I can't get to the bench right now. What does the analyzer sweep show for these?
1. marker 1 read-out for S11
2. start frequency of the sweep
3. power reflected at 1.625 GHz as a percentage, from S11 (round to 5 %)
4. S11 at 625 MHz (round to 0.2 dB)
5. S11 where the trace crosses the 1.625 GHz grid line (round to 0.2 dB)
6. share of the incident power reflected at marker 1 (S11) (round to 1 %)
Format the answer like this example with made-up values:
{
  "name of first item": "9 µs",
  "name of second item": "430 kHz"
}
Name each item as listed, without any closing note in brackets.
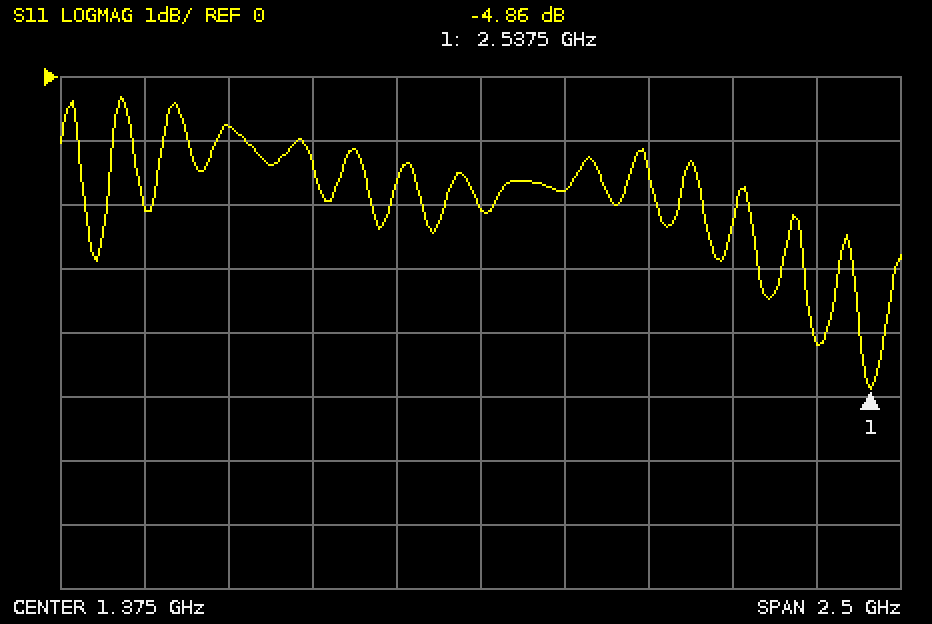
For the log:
{
  "marker 1 read-out for S11": "-4.86 dB",
  "start frequency of the sweep": "125 MHz",
  "power reflected at 1.625 GHz as a percentage, from S11": "65 %",
  "S11 at 625 MHz": "-0.8 dB",
  "S11 where the trace crosses the 1.625 GHz grid line": "-1.8 dB",
  "share of the incident power reflected at marker 1 (S11)": "33 %"
}
